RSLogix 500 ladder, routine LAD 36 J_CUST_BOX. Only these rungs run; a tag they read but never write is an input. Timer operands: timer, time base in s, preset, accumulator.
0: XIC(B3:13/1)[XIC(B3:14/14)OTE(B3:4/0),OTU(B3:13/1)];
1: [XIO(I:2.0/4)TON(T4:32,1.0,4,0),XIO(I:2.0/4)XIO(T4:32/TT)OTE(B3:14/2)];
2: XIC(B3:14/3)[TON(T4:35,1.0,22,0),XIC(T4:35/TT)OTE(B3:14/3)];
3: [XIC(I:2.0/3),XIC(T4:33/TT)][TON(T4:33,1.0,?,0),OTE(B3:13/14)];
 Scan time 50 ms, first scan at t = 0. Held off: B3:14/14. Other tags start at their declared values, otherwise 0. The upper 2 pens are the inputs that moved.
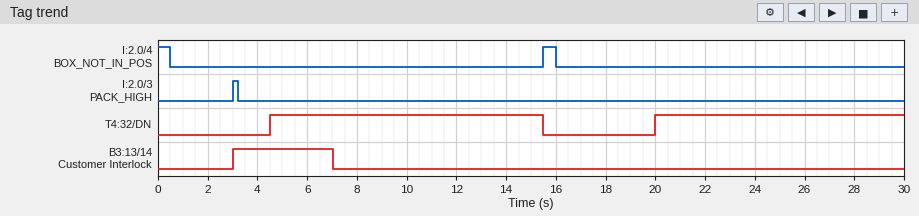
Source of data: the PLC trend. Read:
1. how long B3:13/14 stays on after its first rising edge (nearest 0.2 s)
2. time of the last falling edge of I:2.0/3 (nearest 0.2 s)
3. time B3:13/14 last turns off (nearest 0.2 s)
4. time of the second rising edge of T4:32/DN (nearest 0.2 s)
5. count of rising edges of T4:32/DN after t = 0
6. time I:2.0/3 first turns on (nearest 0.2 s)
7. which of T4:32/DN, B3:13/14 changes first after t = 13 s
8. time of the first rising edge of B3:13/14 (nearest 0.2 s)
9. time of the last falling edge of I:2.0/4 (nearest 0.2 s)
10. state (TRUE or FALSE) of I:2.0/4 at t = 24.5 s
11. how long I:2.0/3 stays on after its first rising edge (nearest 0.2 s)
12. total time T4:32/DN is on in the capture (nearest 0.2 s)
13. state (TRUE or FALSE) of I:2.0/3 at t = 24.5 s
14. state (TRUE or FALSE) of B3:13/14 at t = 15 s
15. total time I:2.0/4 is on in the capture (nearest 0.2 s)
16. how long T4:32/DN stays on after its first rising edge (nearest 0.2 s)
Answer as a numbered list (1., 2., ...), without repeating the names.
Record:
1. 4.0 s
2. 3.2 s
3. 7.0 s
4. 20.0 s
5. 2
6. 3.0 s
7. T4:32/DN
8. 3.0 s
9. 16.0 s
10. FALSE
11. 0.2 s
12. 21.0 s
13. FALSE
14. FALSE
15. 1.0 s
16. 11.0 s
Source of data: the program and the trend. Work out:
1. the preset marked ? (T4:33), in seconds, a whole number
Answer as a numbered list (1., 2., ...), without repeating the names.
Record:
1. 4 s
